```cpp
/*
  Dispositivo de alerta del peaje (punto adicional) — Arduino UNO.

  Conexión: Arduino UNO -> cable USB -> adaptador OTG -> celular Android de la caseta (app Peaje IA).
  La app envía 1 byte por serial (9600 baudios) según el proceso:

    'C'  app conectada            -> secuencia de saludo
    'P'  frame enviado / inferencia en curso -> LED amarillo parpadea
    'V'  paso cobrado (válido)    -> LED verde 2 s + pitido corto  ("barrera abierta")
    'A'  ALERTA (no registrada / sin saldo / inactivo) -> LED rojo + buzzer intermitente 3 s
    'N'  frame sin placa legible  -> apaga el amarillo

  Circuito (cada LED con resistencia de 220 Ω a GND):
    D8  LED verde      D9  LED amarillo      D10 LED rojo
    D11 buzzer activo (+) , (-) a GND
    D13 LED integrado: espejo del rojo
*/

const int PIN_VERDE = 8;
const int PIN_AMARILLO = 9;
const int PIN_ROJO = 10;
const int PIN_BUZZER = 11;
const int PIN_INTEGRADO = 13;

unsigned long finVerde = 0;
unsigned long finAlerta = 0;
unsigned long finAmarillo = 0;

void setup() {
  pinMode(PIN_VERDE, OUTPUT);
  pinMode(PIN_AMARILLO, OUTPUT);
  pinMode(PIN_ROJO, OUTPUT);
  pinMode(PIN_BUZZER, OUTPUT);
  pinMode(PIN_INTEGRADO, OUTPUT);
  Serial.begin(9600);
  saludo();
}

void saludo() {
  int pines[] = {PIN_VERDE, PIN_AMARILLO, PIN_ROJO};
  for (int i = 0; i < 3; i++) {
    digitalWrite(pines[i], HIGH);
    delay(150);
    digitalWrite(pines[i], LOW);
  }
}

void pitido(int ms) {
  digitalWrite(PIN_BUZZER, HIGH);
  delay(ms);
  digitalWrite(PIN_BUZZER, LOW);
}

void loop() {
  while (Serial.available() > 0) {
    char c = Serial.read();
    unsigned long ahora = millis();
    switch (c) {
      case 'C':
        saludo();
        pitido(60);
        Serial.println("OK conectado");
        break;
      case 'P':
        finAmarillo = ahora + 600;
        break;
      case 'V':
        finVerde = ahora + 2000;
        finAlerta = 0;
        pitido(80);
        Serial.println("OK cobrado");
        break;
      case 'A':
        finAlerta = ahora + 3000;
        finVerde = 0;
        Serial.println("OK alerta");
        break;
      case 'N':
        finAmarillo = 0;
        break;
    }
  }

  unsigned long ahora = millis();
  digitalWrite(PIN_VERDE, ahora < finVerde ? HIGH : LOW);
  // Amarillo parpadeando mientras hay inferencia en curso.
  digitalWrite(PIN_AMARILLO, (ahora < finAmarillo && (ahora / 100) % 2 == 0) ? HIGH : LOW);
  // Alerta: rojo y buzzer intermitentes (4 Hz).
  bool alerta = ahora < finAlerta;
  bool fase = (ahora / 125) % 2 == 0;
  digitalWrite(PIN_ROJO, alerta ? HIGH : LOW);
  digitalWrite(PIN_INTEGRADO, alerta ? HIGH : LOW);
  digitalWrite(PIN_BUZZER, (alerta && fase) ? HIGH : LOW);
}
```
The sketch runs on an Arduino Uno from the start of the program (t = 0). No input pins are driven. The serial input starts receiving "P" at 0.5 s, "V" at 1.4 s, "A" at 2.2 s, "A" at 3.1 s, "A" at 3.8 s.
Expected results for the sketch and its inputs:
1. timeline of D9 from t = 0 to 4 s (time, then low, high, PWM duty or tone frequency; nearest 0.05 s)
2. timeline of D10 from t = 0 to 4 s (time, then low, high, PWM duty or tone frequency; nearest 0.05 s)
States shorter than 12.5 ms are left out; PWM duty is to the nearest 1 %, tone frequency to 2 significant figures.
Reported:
0 s low; 0.15 s high; 0.3 s low; 0.6 s high; 0.7 s low; 0.8 s high; 0.9 s low; 1 s high; 1.1 s low
0 s low; 0.3 s high; 0.45 s low; 2.2 s high
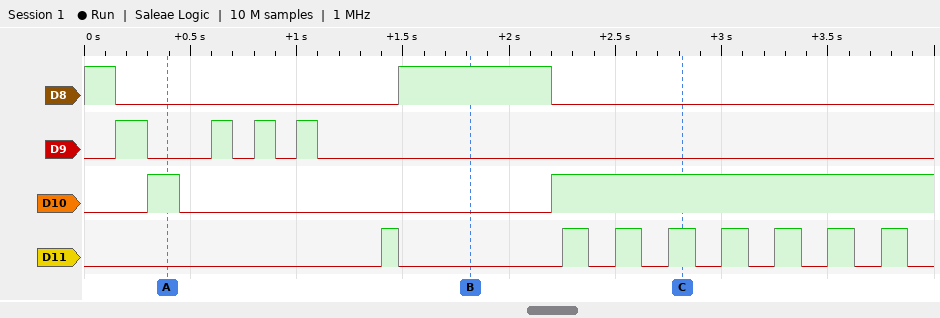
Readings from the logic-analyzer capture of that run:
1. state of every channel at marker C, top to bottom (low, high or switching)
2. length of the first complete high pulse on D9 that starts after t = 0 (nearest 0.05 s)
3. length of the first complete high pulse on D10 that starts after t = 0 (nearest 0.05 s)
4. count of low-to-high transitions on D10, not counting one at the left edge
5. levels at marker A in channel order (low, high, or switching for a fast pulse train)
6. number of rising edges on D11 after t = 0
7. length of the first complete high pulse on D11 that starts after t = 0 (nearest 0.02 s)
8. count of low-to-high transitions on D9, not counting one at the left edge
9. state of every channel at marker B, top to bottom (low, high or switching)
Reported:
D8 low, D9 low, D10 high, D11 high
0.15 s
0.15 s
2
D8 low, D9 low, D10 high, D11 low
8
0.08 s
4
D8 high, D9 low, D10 low, D11 low
